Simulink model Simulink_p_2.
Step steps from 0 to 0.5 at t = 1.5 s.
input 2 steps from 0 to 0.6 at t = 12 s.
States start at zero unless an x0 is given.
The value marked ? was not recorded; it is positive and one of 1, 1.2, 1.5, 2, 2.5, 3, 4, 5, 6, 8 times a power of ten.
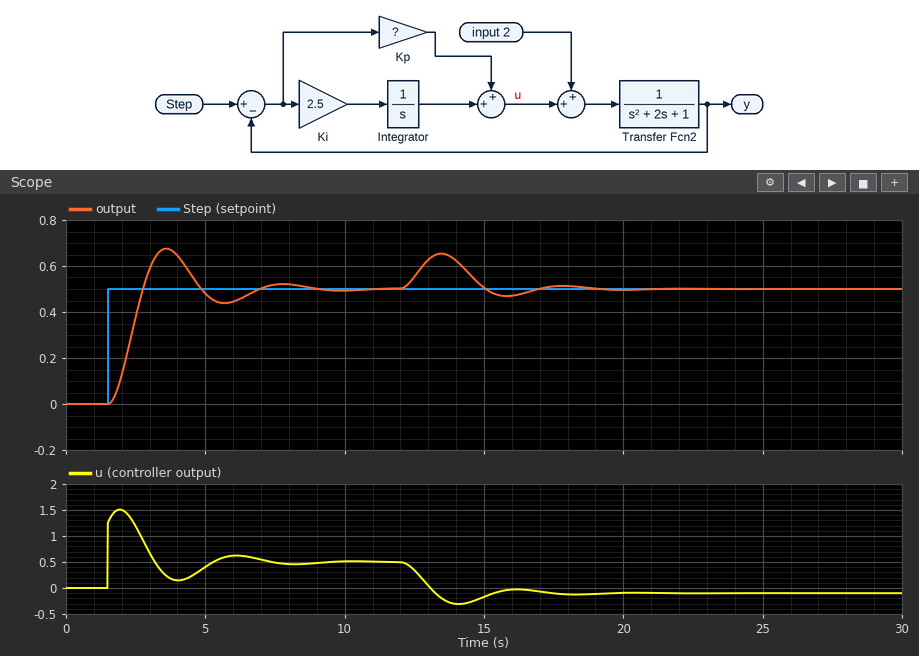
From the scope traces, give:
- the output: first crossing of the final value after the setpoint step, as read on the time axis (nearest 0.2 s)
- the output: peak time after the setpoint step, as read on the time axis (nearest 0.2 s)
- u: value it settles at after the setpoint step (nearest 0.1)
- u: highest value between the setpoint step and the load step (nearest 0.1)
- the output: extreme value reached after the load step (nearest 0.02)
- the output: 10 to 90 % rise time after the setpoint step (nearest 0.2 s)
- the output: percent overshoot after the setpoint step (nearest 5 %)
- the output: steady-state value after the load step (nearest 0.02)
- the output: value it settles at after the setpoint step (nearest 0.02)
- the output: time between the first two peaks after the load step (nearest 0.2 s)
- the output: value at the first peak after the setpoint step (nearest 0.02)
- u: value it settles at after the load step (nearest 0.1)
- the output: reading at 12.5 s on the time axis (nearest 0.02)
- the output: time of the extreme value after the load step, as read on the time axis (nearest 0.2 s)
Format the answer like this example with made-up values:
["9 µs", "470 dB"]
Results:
["2.8 s", "3.6 s", "0.5", "1.5", "0.66", "0.8 s", "35 %", "0.50", "0.50", "4.4 s", "0.68", "-0.1", "0.56", "13.4 s"]
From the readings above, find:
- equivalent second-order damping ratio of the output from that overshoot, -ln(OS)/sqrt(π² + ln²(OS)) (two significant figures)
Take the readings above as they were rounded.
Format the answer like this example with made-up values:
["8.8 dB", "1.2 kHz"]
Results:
["0.32"]
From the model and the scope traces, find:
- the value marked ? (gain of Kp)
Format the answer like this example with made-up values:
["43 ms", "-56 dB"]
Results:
["2.5"]
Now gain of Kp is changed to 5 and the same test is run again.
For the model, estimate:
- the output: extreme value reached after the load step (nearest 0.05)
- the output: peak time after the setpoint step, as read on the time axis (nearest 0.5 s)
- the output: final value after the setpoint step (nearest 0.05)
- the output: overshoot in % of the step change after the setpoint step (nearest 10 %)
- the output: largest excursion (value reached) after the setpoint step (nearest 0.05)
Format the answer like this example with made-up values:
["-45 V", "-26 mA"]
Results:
["0.60", "3.0 s", "0.50", "30 %", "0.65"]
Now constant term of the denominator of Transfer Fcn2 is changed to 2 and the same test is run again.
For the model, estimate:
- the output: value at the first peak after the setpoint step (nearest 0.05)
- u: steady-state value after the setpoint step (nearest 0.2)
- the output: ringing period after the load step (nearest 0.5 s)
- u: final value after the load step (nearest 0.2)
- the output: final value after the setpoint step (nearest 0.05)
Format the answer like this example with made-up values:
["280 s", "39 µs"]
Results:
["0.55", "1.0", "3.5 s", "0.4", "0.50"]
